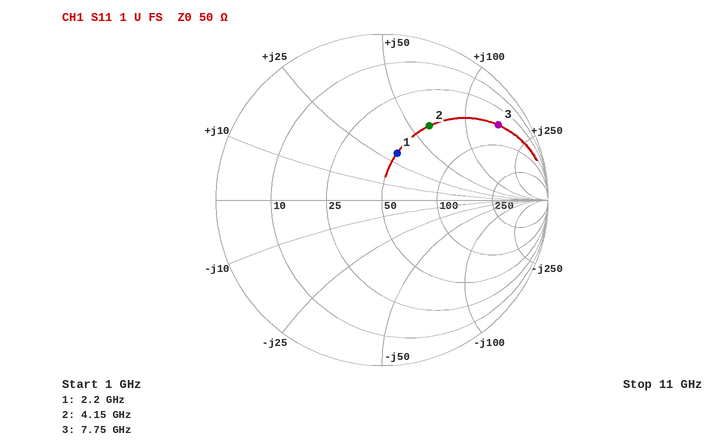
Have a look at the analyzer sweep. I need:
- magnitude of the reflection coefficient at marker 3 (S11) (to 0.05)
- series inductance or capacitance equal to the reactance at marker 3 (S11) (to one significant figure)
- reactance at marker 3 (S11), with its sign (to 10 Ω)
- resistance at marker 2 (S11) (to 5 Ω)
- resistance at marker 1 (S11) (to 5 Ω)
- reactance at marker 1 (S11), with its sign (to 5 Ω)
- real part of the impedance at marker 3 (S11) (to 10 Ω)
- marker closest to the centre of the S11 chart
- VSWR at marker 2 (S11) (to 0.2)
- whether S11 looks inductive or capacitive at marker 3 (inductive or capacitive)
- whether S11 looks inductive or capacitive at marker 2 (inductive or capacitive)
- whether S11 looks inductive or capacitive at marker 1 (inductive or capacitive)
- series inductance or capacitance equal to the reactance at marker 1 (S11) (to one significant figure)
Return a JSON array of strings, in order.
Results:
["0.85", "3 nH", "+150 Ω", "50 Ω", "50 Ω", "+30 Ω", "50 Ω", "marker 1", "3.2", "inductive", "inductive", "inductive", "2 nH"]
